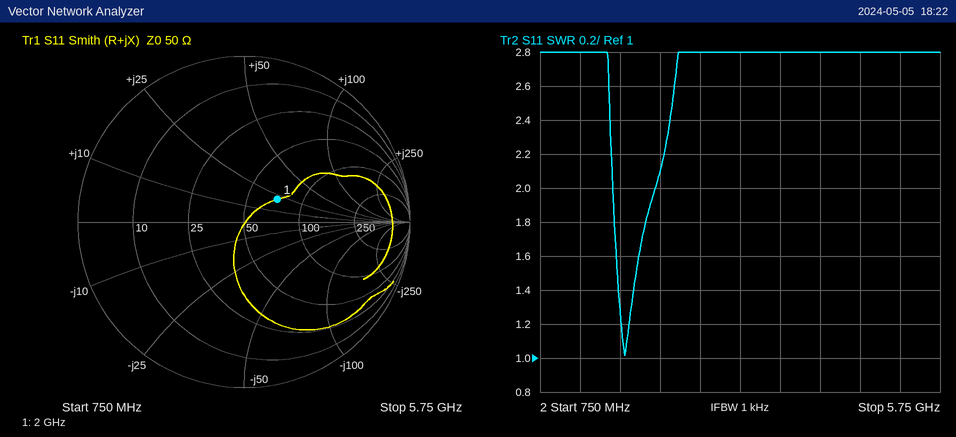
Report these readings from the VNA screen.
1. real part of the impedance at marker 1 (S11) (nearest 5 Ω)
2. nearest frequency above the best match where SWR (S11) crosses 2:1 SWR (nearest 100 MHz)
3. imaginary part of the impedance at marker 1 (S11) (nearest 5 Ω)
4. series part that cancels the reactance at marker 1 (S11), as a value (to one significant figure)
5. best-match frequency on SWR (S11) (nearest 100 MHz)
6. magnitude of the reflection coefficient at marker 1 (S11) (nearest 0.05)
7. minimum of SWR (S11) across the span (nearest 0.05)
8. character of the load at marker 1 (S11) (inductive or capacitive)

70 Ω
2.2 GHz
+20 Ω
4 pF
1.8 GHz
0.25
1.00
inductive
